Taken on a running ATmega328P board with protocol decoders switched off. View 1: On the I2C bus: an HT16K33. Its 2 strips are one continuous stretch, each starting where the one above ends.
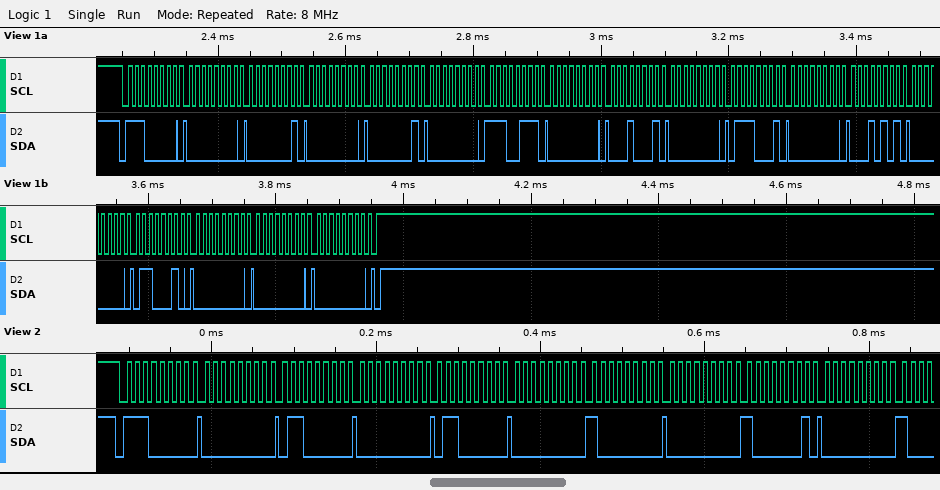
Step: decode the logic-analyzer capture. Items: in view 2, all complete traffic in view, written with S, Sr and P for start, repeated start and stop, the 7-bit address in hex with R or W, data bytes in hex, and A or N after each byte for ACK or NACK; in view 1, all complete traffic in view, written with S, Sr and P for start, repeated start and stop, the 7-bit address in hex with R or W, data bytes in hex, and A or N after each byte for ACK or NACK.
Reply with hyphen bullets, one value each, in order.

- S 70W A 00 A 60 A 00 A 60 A 00 A 80 A 00 A 81 A 00 A
- S 70W A 00 A 01 A 00 A 01 A 00 A E7 A 00 A 11 A 00 A 71 A 00 A 15 A 00 A 62 A 00 A 00 A 00 A P
